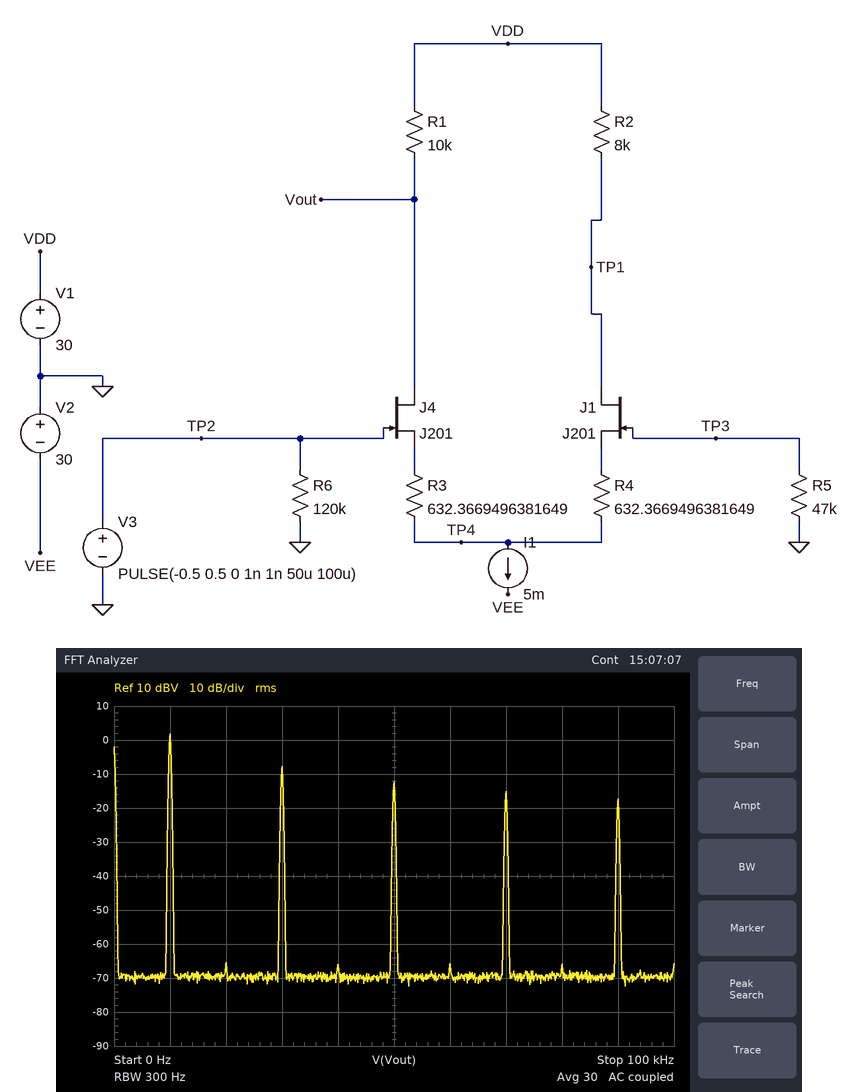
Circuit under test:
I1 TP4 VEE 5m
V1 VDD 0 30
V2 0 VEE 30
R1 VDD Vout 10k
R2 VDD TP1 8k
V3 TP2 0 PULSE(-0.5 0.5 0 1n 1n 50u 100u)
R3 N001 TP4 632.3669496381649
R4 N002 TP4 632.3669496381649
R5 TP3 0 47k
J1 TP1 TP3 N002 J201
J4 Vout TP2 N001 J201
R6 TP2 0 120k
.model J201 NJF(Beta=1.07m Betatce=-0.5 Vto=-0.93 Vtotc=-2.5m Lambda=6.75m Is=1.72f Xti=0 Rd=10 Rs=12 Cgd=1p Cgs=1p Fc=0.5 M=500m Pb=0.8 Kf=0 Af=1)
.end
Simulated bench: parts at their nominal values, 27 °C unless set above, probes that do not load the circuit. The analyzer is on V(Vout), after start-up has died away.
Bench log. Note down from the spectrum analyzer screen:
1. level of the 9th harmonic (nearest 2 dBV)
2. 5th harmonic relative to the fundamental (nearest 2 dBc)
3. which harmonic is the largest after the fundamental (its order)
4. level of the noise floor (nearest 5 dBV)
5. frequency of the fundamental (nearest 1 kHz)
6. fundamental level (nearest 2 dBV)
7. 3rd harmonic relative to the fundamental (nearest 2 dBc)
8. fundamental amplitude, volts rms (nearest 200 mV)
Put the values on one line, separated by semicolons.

-18 dBV; -14 dBc; 3; -70 dBV; 10 kHz; 2 dBV; -10 dBc; 1.2 V
